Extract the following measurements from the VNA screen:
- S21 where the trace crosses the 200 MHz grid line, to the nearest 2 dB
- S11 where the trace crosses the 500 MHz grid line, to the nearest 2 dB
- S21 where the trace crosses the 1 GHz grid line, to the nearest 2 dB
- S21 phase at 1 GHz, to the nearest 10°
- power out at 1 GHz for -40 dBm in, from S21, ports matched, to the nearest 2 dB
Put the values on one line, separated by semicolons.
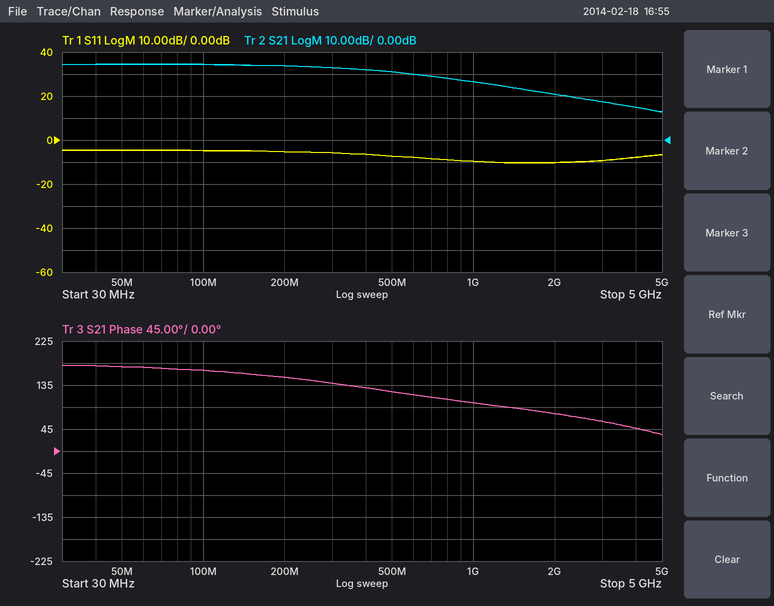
34 dB; -8 dB; 26 dB; 100°; -14 dBm
